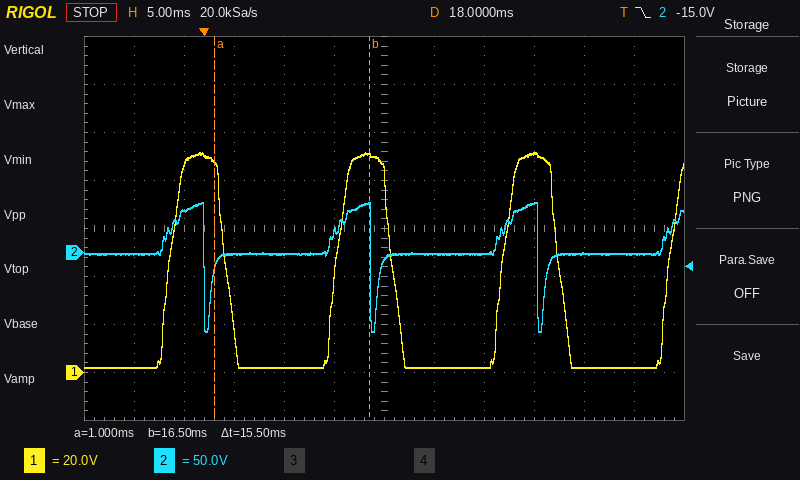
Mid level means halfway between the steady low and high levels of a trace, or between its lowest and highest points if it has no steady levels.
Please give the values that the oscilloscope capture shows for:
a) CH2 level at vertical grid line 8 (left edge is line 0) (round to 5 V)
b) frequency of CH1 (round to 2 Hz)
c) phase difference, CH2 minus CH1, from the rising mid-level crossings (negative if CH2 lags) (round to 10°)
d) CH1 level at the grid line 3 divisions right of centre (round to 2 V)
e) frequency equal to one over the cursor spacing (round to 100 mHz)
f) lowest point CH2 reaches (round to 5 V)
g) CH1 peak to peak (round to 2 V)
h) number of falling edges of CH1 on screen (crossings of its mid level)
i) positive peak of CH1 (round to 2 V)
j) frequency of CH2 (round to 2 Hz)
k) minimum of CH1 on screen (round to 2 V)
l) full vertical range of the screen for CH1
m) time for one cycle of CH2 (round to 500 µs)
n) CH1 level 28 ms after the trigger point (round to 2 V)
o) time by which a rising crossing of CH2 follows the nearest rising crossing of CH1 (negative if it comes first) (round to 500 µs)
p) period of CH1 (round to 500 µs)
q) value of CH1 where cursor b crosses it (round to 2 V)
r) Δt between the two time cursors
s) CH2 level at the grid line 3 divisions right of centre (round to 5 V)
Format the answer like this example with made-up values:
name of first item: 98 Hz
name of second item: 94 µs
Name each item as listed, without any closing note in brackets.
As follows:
CH2 level at vertical grid line 8 (left edge is line 0): 0 V
frequency of CH1: 60 Hz
phase difference, CH2 minus CH1, from the rising mid-level crossings (negative if CH2 lags): -100°
CH1 level at the grid line 3 divisions right of centre: 92 V
frequency equal to one over the cursor spacing: 64.5 Hz
lowest point CH2 reaches: -80 V
CH1 peak to peak: 90 V
number of falling edges of CH1 on screen: 3
positive peak of CH1: 92 V
frequency of CH2: 60 Hz
minimum of CH1 on screen: 2 V
full vertical range of the screen for CH1: 160 V
time for one cycle of CH2: 16.5 ms
CH1 level 28 ms after the trigger point: 2 V
time by which a rising crossing of CH2 follows the nearest rising crossing of CH1 (negative if it comes first): +4.5 ms
period of CH1: 16.5 ms
value of CH1 where cursor b crosses it: 90 V
Δt between the two time cursors: 15.5 ms
CH2 level at the grid line 3 divisions right of centre: 50 V
